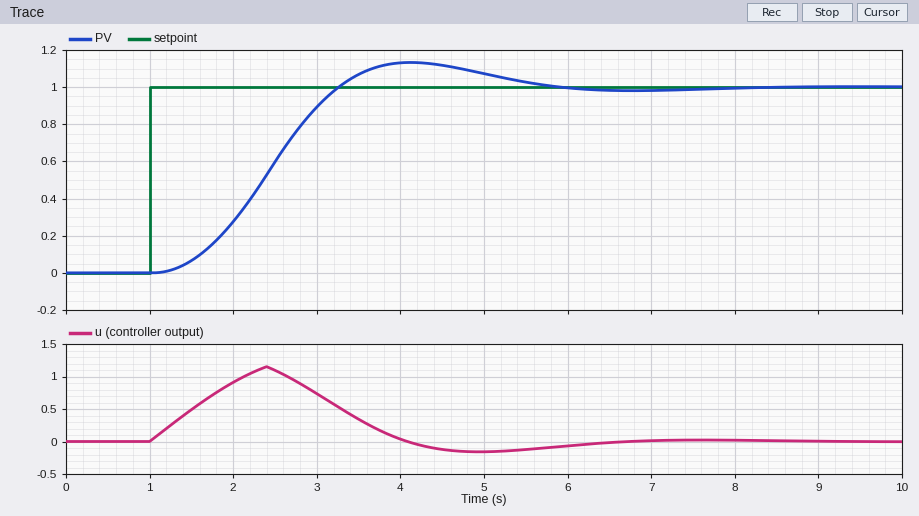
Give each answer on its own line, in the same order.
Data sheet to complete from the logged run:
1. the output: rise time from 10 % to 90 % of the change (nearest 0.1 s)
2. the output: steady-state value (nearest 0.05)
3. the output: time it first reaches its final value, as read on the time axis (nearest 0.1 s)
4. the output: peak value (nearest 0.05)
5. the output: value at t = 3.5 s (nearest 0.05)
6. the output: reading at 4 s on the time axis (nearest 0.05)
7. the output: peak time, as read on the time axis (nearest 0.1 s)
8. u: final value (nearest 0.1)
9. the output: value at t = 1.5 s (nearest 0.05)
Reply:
1.4 s
1.00
3.3 s
1.15
1.05
1.15
4.1 s
0.0
0.05
